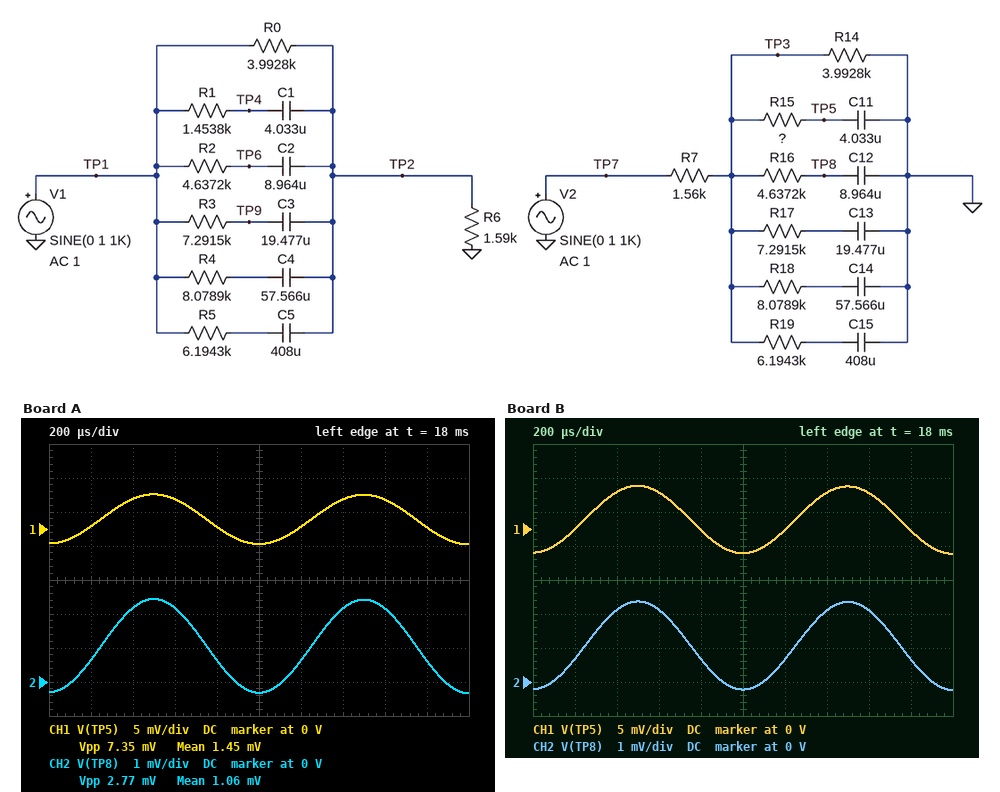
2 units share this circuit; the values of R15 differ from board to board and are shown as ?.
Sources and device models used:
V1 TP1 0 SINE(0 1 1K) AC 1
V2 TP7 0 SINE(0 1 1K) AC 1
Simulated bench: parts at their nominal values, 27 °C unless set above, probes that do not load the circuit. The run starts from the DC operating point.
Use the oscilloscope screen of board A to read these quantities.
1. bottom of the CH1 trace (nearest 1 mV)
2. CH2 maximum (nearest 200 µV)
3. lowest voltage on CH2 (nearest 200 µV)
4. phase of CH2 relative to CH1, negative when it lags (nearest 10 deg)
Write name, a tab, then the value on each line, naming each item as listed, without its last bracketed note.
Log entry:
bottom of the CH1 trace	-2 mV
CH2 maximum	2.4 mV
lowest voltage on CH2	-400 µV
phase of CH2 relative to CH1, negative when it lags	0 deg
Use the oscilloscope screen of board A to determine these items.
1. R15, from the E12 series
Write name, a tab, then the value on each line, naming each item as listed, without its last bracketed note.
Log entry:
R15, from the E12 series	3.9 kΩ
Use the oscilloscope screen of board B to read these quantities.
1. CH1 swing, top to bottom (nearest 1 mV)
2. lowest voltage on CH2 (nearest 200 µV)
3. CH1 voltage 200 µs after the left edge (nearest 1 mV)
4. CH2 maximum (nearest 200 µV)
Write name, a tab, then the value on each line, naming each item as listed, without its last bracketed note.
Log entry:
CH1 swing, top to bottom	10 mV
lowest voltage on CH2	-200 µV
CH1 voltage 200 µs after the left edge	0 V
CH2 maximum	2.4 mV
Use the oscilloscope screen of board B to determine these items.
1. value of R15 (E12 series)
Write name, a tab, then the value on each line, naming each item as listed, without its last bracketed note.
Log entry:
value of R15	2.7 kΩ
